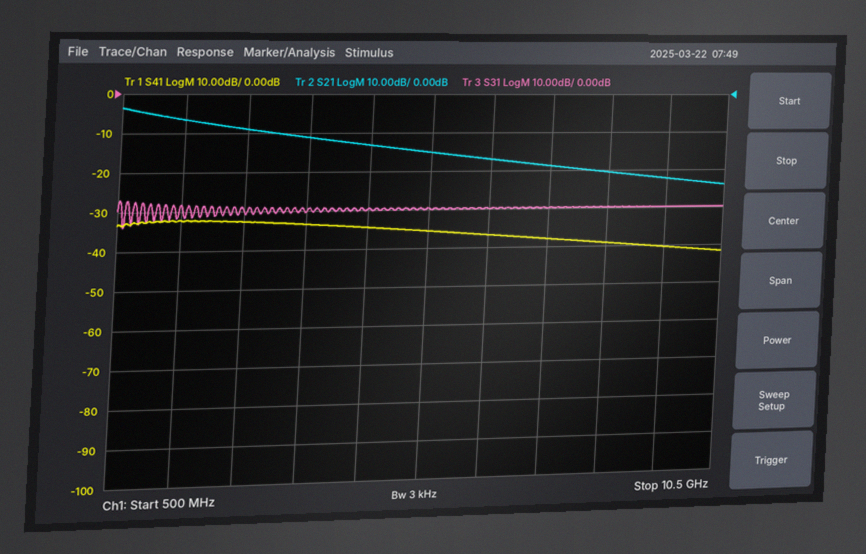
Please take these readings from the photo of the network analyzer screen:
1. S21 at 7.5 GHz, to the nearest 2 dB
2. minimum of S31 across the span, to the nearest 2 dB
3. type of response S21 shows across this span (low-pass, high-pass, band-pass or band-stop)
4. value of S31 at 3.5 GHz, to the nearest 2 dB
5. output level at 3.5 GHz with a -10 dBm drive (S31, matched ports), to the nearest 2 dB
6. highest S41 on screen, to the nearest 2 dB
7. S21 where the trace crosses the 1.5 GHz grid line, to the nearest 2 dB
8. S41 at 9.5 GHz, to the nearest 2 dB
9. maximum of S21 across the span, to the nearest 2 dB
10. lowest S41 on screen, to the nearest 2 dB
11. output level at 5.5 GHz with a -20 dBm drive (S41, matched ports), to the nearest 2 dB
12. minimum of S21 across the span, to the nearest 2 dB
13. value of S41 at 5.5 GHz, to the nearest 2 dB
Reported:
-18 dB
-34 dB
low-pass
-30 dB
-40 dBm
-32 dB
-6 dB
-40 dB
-4 dB
-42 dB
-56 dBm
-24 dB
-36 dB
